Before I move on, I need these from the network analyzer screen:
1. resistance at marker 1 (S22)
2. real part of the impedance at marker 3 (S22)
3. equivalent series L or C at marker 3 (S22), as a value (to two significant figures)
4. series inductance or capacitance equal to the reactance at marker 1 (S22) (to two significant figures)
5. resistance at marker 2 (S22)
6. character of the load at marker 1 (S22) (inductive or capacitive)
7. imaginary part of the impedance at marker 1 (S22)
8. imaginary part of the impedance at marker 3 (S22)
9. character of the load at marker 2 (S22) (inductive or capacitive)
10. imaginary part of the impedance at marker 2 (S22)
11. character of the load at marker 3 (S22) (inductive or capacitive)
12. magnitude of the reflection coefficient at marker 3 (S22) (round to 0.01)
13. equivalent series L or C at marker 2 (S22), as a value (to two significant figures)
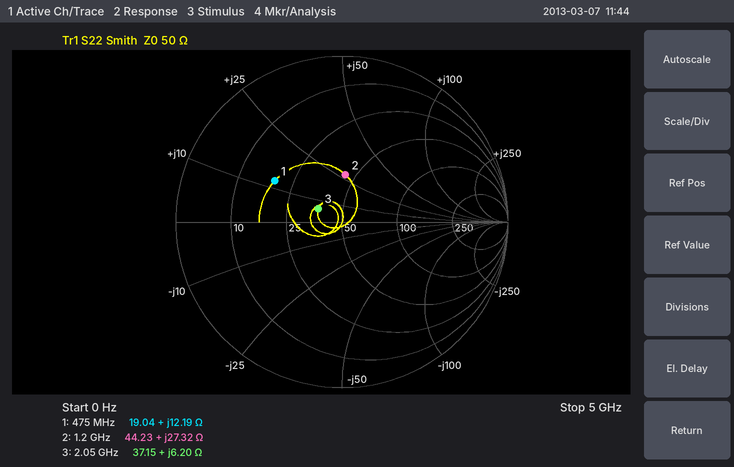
19.04 Ω
37.15 Ω
480 pH
4.1 nH
44.23 Ω
inductive
+12.19 Ω
+6.20 Ω
inductive
+27.32 Ω
inductive
0.16
3.6 nH
